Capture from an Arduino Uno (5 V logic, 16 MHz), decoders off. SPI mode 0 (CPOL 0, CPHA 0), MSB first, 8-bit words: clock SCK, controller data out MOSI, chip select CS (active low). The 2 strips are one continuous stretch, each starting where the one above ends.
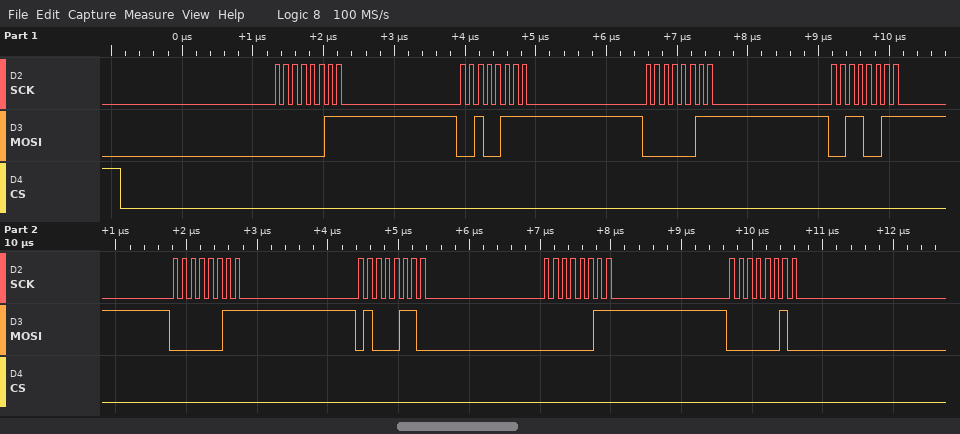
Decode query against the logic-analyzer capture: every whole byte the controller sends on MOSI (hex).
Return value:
03 27 03 33 03 46 03 02
